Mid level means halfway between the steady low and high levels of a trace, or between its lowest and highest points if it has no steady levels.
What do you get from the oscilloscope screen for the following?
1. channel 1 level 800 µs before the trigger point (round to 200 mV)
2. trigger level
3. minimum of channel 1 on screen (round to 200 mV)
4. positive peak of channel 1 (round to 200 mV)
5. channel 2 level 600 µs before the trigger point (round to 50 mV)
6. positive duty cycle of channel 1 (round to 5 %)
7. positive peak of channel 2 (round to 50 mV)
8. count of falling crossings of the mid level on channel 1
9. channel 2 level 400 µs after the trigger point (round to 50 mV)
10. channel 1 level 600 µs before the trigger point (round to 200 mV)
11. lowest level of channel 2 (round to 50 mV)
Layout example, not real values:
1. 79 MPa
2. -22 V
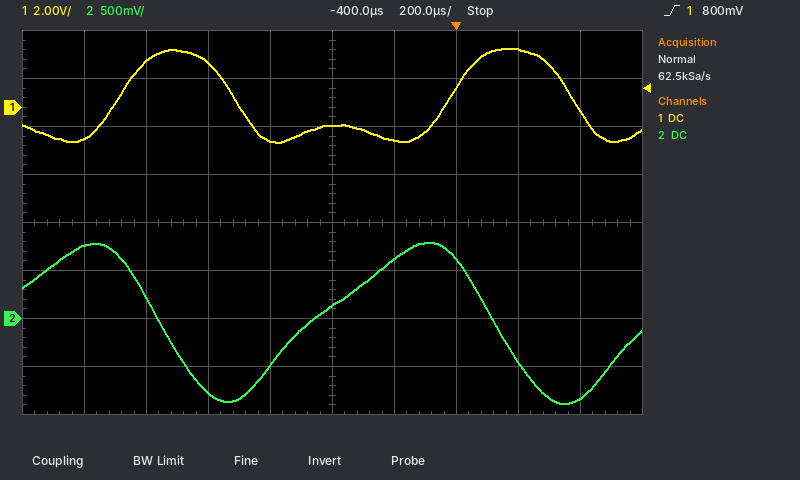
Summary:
1. 1.8 V
2. 800 mV
3. -1.4 V
4. 2.4 V
5. -500 mV
6. 35 %
7. 800 mV
8. 2
9. -850 mV
10. -1.4 V
11. -900 mV
